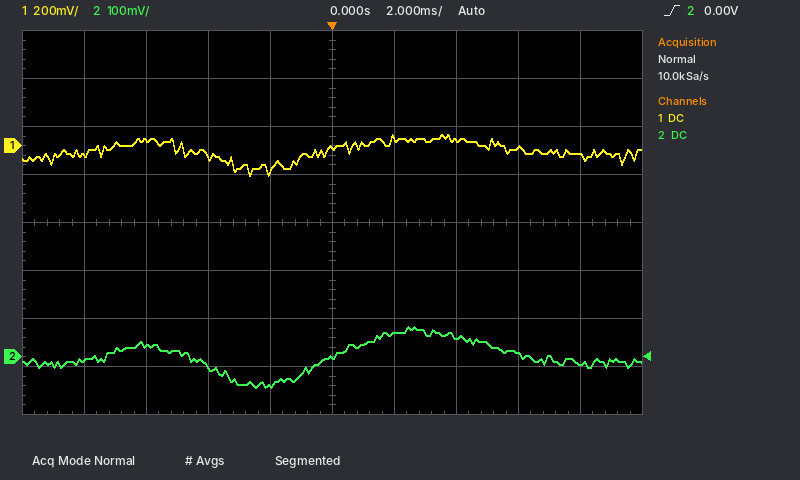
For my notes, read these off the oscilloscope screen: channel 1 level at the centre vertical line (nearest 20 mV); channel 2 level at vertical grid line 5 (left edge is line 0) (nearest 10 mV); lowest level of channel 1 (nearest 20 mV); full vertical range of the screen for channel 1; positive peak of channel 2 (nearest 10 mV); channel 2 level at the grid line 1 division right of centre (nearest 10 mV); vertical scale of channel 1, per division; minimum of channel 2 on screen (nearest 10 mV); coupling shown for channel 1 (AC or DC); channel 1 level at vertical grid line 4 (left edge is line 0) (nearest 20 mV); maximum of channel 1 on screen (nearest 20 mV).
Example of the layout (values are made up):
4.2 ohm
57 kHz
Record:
0 mV
0 mV
-120 mV
1.6 V
60 mV
50 mV
200 mV
-60 mV
DC
-100 mV
40 mV
